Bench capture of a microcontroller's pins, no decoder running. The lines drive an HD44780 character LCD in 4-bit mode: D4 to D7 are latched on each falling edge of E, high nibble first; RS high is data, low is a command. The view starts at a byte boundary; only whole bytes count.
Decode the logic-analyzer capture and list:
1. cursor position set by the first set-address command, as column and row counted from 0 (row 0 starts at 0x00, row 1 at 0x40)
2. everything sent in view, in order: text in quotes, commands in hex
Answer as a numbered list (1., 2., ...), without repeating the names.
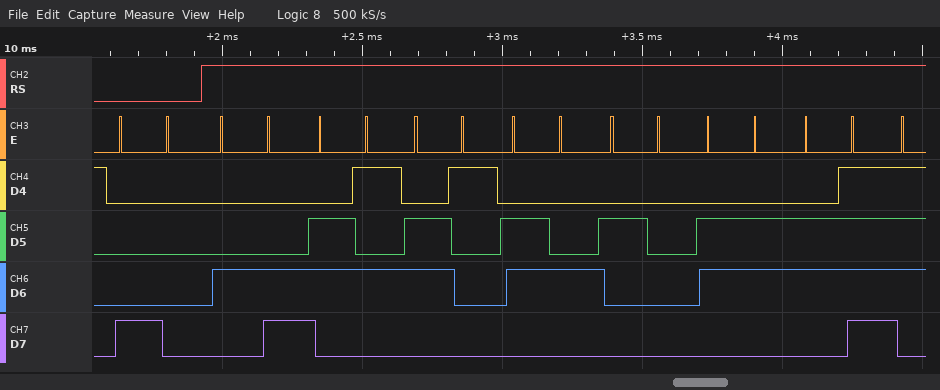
1. column 0, row 0
2. 0x80 "Lead fo"
